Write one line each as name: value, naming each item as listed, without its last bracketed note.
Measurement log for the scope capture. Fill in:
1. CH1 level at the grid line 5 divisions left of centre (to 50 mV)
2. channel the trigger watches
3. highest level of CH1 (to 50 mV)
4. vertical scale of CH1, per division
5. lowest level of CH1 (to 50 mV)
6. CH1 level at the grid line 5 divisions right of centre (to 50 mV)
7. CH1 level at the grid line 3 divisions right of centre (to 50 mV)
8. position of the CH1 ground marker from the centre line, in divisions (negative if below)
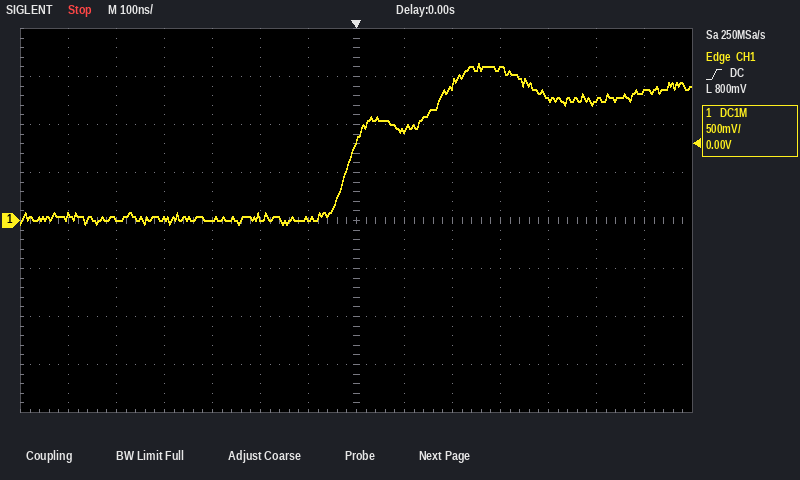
CH1 level at the grid line 5 divisions left of centre: 0 mV
channel the trigger watches: CH1
highest level of CH1: 1.65 V
vertical scale of CH1, per division: 500 mV
lowest level of CH1: -50 mV
CH1 level at the grid line 5 divisions right of centre: 1.25 V
CH1 level at the grid line 3 divisions right of centre: 1.60 V
position of the CH1 ground marker from the centre line, in divisions: 0.0 div
